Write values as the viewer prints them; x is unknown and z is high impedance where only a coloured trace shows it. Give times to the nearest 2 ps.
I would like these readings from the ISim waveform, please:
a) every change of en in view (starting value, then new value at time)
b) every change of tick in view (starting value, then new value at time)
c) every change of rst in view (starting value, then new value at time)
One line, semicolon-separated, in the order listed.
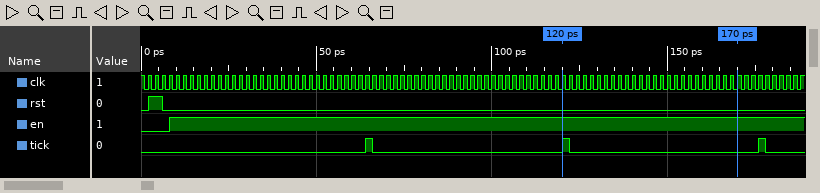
0, 1 at 8 ps; 0, 1 at 64 ps, 0 at 66 ps, 1 at 120 ps, 0 at 122 ps, 1 at 176 ps, 0 at 178 ps; 0, 1 at 2 ps, 0 at 6 ps
